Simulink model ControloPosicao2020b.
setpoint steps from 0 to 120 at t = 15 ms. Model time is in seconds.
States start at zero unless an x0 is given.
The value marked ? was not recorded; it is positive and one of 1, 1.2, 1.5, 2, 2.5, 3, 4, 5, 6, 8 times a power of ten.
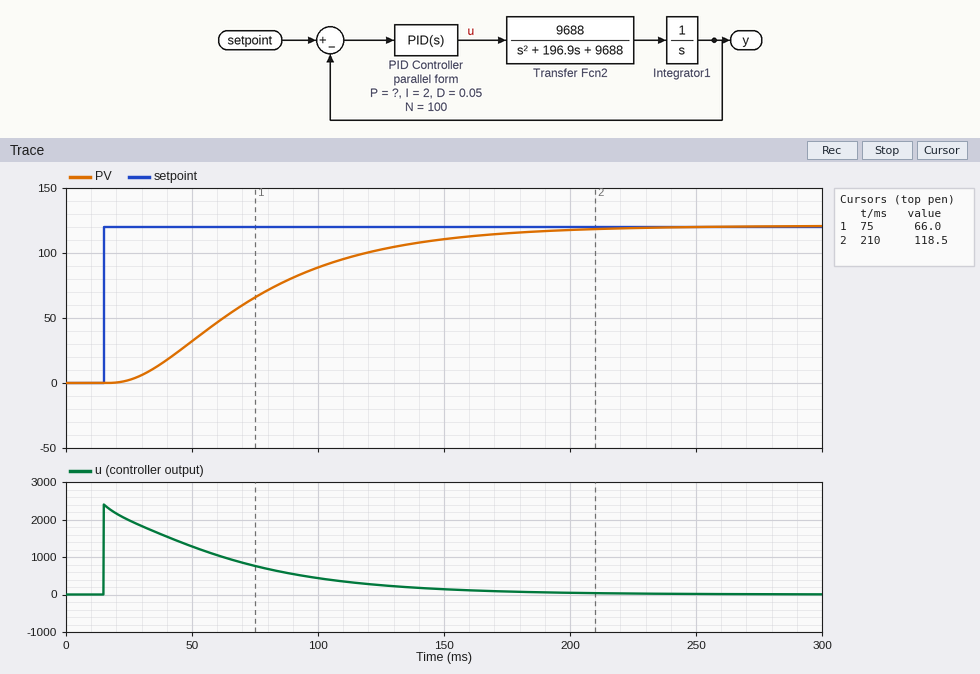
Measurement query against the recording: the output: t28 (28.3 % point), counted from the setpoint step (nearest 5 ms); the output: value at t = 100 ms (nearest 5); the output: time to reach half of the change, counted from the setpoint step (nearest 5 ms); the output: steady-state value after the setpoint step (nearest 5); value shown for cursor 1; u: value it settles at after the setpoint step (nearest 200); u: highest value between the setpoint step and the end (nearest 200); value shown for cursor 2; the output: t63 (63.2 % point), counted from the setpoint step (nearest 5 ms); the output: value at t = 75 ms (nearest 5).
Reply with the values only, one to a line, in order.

35 ms
90
55 ms
120
66.0
0
2400
118.5
70 ms
65
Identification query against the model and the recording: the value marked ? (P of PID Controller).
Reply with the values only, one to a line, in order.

15
